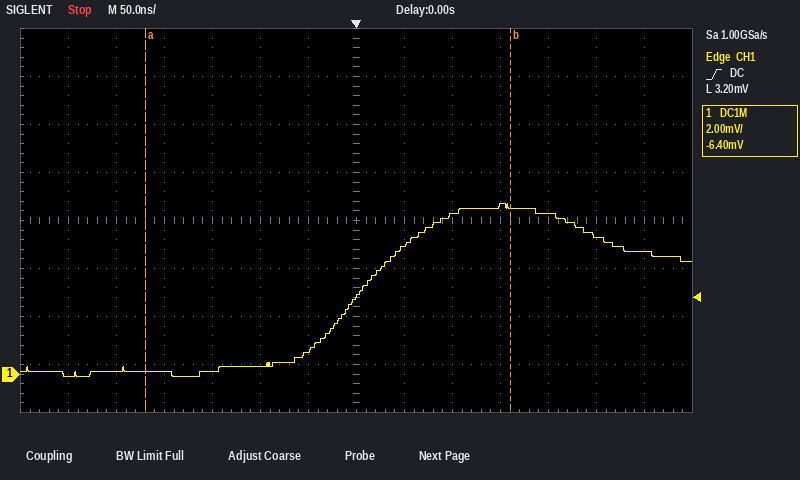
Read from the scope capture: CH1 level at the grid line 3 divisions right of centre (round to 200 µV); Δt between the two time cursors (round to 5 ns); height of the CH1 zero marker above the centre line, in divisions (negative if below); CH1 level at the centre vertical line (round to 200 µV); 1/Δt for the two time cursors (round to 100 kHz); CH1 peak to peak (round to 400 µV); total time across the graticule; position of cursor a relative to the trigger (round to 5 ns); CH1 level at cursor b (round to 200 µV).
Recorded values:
7.0 mV
380 ns
-3.2 div
3.2 mV
2.6 MHz
7.2 mV
700 ns
-220 ns
7.0 mV
